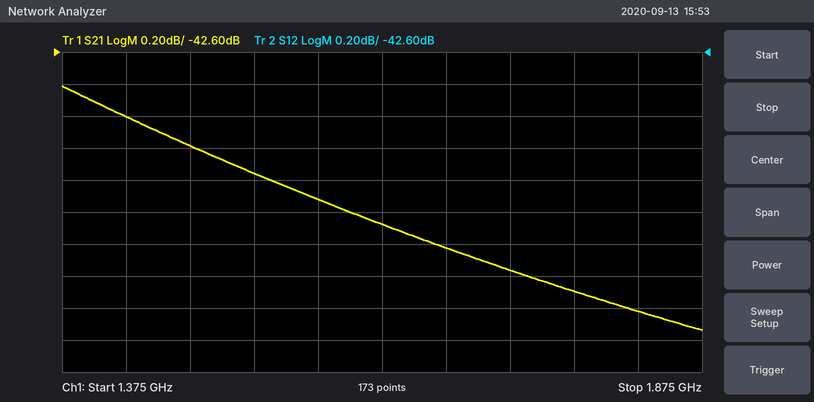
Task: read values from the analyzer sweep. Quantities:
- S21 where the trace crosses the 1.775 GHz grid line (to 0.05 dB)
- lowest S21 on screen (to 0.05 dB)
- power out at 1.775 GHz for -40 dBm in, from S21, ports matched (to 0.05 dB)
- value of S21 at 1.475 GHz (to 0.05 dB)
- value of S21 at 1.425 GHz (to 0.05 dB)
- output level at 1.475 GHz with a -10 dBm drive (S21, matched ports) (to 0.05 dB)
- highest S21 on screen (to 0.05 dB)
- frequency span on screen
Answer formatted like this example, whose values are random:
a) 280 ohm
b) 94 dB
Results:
a) -44.10 dB
b) -44.35 dB
c) -84.10 dBm
d) -43.20 dB
e) -43.00 dB
f) -53.20 dBm
g) -42.80 dB
h) 500 MHz
